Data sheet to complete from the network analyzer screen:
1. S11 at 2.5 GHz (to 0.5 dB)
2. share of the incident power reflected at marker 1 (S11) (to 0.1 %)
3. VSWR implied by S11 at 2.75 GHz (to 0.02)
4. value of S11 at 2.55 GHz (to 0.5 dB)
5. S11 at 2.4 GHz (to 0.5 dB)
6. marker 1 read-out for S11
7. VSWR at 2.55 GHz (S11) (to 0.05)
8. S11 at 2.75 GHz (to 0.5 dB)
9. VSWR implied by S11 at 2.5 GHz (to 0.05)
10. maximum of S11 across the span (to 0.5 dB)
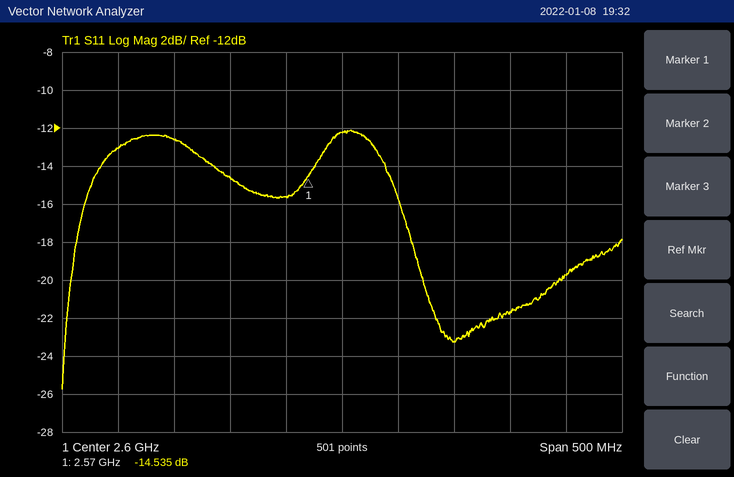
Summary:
-14.5 dB
3.5 %
1.18
-15.5 dB
-13.0 dB
-14.535 dB
1.40
-21.5 dB
1.45
-12.0 dB
